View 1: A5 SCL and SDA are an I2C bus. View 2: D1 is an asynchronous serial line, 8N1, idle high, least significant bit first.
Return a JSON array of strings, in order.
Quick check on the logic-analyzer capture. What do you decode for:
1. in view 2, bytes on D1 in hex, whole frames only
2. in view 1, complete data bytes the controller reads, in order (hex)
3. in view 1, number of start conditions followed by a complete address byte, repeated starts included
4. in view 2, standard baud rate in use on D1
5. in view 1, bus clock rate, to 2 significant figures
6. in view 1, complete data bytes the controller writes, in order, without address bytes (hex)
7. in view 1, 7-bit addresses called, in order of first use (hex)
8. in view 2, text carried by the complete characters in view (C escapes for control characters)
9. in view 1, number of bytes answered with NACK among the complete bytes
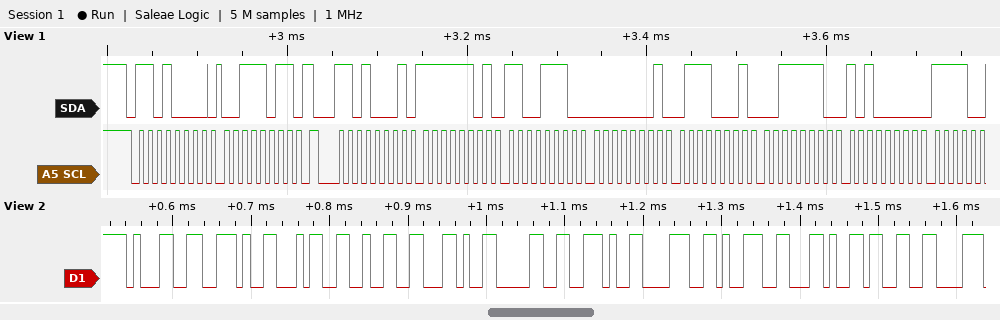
["31 2E 34 32 2C 30 2E 38 39 2C 33", "FD CE 01 71 3E A0", "2", "115200 baud", "100 kHz", "3B", "0x68", "\"1.42,0.89,3\"", "0"]
